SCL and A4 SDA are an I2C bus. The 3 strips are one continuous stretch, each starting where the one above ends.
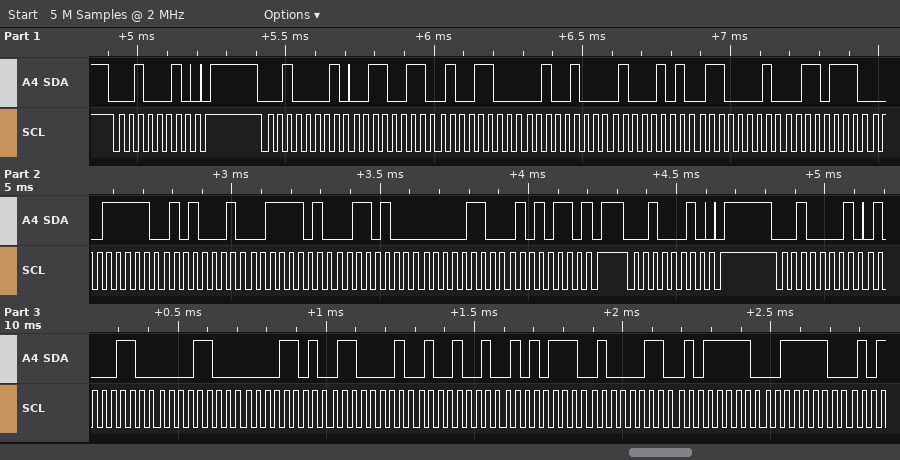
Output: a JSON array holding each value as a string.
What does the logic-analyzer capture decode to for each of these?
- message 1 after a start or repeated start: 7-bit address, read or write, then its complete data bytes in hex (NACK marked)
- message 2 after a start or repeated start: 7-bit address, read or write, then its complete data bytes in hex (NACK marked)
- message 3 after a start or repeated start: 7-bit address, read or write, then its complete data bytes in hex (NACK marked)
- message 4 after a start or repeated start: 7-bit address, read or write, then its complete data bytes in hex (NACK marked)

["0x11 write", "0x10 read: 33 4C 24 45 61 37 1F 51 3D 34 06 56 NACK", "0x11 write", "0x10 read: 46 0C 0D 61 49 57 43 5F 3E"]
